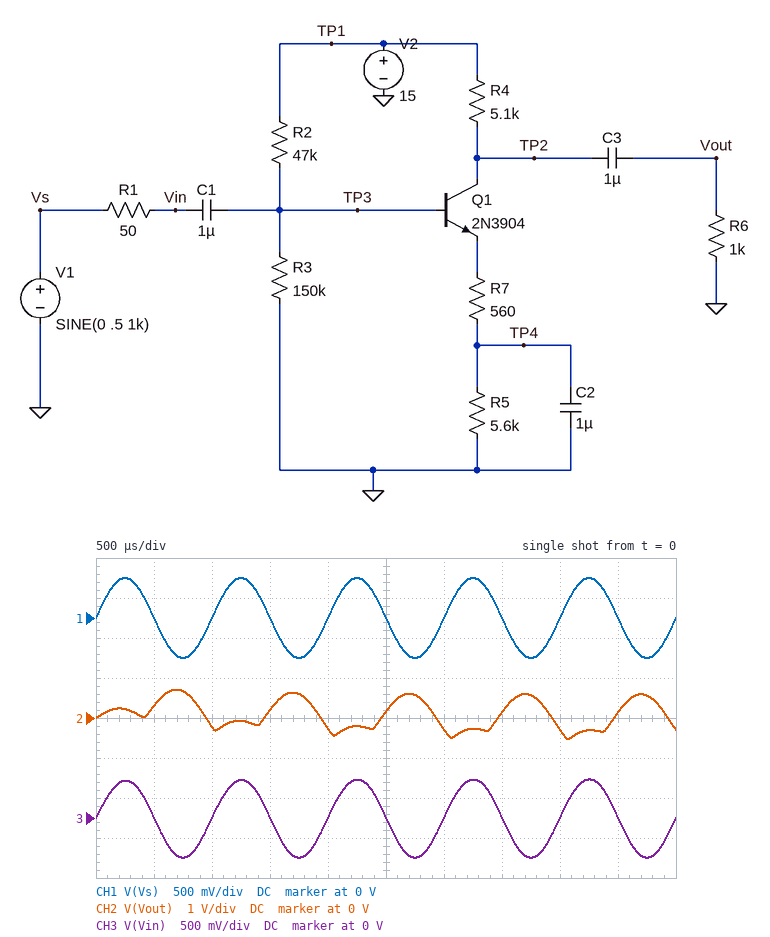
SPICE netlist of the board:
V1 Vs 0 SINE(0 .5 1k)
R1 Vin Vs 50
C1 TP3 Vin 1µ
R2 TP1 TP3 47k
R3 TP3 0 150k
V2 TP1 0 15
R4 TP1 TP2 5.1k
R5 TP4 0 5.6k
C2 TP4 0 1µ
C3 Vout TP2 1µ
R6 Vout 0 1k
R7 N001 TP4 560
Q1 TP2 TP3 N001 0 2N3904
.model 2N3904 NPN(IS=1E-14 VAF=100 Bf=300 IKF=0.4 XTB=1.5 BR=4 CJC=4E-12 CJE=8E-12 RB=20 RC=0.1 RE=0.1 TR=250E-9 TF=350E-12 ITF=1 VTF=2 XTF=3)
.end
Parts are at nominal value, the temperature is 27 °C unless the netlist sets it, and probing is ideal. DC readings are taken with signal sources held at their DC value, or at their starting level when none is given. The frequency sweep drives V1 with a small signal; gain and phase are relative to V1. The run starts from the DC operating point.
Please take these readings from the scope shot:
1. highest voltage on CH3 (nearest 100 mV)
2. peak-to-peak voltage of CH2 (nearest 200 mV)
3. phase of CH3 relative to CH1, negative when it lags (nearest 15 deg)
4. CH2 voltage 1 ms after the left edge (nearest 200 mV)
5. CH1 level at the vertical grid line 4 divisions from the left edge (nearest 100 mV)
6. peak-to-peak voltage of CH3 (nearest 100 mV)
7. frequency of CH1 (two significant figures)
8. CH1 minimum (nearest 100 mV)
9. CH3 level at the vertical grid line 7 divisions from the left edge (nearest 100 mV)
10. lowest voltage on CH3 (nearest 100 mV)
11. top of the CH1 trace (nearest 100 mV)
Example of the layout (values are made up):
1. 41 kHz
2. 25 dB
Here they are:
1. 500 mV
2. 1.2 V
3. 0 deg
4. -200 mV
5. 0 V
6. 1.0 V
7. 1.0 kHz
8. -500 mV
9. 0 V
10. -500 mV
11. 500 mV
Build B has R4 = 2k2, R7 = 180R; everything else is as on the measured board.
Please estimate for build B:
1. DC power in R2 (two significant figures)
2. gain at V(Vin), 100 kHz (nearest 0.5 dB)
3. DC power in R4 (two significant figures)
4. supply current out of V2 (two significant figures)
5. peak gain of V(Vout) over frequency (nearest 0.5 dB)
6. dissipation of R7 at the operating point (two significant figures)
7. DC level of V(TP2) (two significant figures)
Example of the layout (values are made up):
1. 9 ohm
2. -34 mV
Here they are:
1. 310 µW
2. 0 dB
3. 7.3 mW
4. 1.9 mA
5. 11.0 dB
6. 600 µW
7. 11 V
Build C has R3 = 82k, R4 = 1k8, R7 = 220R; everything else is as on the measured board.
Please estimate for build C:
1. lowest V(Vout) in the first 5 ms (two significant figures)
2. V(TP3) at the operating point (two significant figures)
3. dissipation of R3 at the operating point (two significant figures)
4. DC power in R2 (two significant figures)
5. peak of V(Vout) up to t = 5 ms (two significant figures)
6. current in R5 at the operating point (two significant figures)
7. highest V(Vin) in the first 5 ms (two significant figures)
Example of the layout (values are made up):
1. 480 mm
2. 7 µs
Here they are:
1. -1.1 V
2. 9.4 V
3. 1.1 mW
4. 670 µW
5. 960 mV
6. 1.5 mA
7. 500 mV
